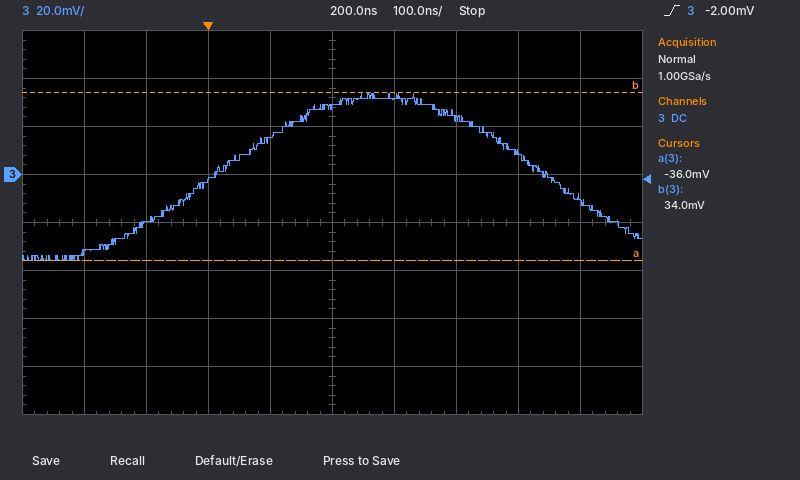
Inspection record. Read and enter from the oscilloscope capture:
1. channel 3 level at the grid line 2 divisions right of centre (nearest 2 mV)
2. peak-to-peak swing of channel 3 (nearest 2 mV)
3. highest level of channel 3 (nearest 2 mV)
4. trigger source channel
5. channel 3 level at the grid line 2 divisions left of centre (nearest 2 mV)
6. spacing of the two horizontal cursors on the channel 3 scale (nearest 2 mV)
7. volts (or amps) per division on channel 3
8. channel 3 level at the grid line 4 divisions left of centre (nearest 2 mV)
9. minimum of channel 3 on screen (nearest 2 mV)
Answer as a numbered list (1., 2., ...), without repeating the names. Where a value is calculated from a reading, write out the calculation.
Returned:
1. 24 mV
2. 34 mV − (-36 mV) = 70 mV
3. 34 mV
4. channel 3
5. -2 mV
6. 70 mV
7. 20 mV
8. -32 mV
9. -36 mV
